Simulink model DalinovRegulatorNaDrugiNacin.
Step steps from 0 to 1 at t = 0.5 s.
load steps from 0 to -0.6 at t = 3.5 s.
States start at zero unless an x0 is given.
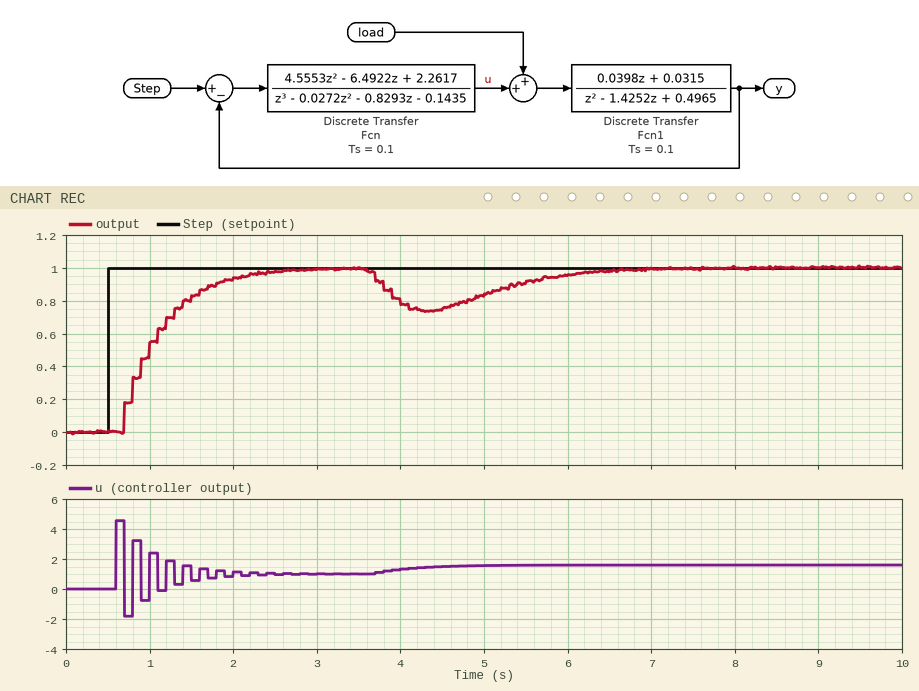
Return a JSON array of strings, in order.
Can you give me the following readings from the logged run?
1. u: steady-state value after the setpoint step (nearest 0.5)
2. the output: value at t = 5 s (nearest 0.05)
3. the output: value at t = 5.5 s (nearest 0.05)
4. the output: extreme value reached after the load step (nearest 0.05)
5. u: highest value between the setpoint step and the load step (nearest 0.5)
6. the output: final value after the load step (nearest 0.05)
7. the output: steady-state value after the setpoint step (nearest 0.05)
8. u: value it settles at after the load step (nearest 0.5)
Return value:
["1.0", "0.85", "0.90", "0.75", "4.5", "1.00", "1.00", "1.5"]
